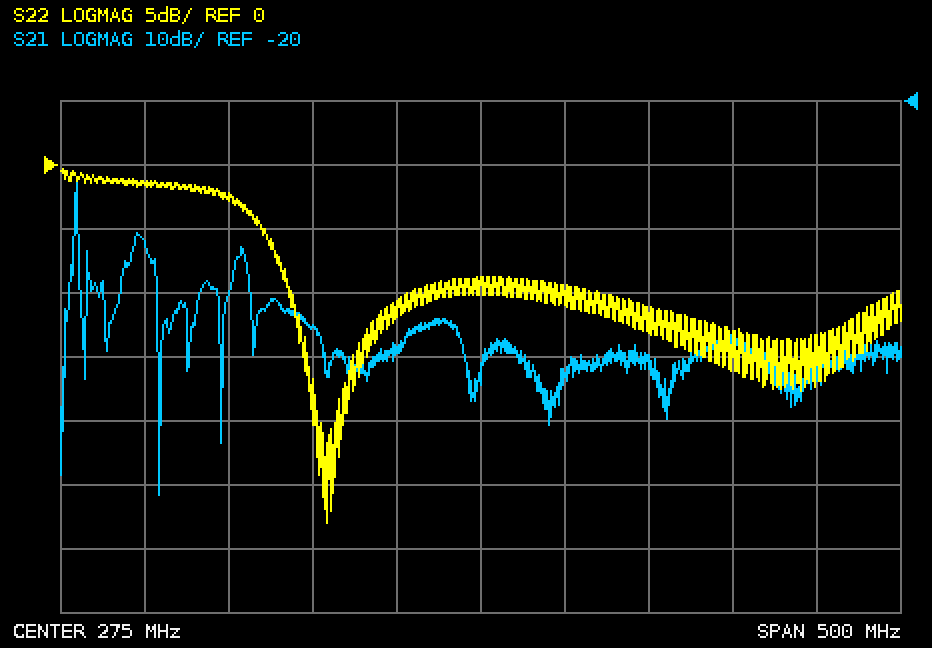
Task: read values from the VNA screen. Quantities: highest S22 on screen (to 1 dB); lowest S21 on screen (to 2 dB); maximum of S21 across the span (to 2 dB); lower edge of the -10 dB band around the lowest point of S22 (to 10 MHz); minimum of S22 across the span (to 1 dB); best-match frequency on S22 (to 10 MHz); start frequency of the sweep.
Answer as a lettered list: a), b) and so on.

a) 0 dB
b) -82 dB
c) -32 dB
d) 160 MHz
e) -28 dB
f) 180 MHz
g) 25 MHz
